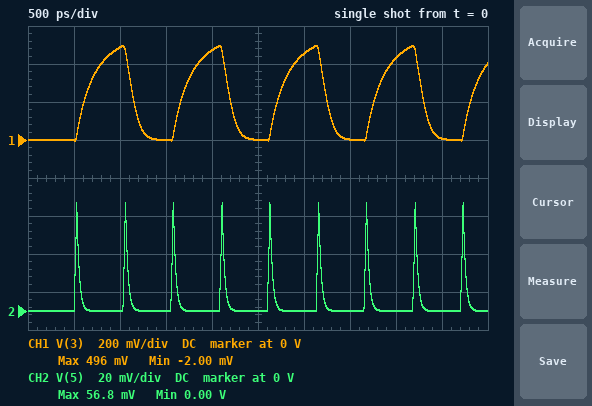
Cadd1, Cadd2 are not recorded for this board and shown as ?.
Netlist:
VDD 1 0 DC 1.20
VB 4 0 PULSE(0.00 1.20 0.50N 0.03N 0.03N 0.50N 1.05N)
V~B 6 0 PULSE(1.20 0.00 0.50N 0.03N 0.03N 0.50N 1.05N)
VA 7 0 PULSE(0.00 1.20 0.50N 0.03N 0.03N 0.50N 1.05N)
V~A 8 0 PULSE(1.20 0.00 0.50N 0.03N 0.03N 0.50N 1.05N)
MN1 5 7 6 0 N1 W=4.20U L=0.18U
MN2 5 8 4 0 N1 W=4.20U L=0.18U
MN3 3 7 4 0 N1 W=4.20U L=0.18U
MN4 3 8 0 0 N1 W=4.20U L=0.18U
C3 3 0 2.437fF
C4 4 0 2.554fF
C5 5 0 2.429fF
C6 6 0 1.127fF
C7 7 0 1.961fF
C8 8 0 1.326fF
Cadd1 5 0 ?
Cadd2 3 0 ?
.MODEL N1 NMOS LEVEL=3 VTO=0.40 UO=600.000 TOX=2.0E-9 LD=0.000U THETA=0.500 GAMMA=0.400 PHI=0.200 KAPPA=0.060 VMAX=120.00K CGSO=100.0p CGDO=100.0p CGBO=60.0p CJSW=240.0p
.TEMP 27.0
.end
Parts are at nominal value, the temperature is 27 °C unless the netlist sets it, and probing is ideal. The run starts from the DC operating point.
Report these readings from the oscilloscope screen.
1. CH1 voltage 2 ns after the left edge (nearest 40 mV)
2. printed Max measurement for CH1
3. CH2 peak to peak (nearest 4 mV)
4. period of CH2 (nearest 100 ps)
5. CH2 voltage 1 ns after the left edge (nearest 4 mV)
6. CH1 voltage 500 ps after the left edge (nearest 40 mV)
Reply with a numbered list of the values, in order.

1. 480 mV
2. 496 mV
3. 56 mV
4. 500 ps
5. 0 V
6. 0 V
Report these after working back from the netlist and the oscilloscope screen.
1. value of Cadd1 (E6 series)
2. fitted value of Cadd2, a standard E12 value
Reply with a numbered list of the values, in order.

1. 330 fF
2. 680 fF
